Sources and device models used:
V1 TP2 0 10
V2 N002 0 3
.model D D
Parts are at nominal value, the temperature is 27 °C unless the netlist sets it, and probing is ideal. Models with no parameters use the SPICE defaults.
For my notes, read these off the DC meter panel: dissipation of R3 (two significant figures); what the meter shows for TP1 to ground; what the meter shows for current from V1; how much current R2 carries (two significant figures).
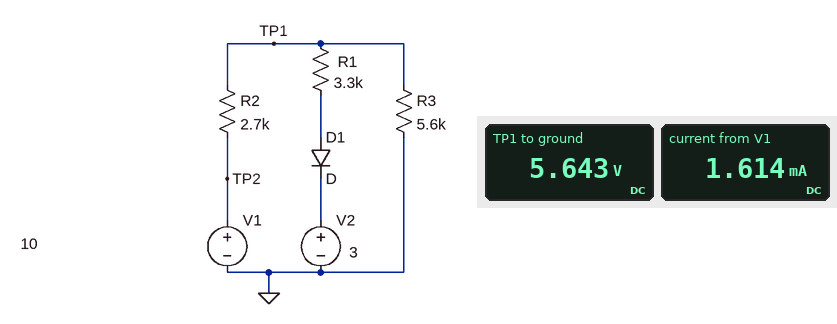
5.7 mW
5.643 V
1.614 mA
1.6 mA
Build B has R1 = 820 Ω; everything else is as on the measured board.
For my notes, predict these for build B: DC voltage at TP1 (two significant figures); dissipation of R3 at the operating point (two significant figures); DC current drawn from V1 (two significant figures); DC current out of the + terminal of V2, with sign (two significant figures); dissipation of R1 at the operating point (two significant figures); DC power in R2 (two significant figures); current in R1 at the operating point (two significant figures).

4.6 V
3.8 mW
2.0 mA
-1.2 mA
1.1 mW
11 mW
1.2 mA
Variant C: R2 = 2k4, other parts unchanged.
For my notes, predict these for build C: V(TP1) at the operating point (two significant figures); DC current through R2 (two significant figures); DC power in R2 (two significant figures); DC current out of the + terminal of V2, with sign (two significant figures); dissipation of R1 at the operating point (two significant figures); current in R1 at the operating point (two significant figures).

5.9 V
1.7 mA
7.1 mW
-670 µA
1.5 mW
670 µA
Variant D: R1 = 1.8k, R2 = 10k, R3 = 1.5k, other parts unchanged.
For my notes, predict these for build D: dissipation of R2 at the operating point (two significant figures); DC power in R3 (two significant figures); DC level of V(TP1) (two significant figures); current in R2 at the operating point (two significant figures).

7.6 mW
1.1 mW
1.3 V
870 µA
